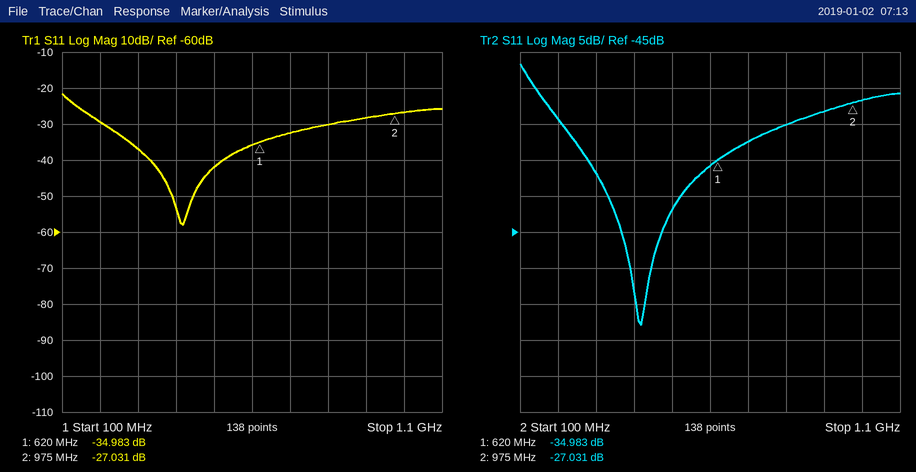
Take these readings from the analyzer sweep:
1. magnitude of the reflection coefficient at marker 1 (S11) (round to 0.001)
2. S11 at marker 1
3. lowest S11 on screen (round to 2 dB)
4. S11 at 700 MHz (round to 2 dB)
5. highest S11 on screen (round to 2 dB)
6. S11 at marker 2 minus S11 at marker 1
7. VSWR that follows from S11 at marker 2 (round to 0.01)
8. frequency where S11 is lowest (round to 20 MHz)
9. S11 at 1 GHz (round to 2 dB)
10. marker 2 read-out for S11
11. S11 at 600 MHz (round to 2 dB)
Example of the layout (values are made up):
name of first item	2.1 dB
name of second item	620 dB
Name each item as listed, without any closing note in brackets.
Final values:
magnitude of the reflection coefficient at marker 1 (S11)	0.018
S11 at marker 1	-34.983 dB
lowest S11 on screen	-58 dB
S11 at 700 MHz	-32 dB
highest S11 on screen	-22 dB
S11 at marker 2 minus S11 at marker 1	7.952 dB
VSWR that follows from S11 at marker 2	1.09
frequency where S11 is lowest	420 MHz
S11 at 1 GHz	-26 dB
marker 2 read-out for S11	-27.031 dB
S11 at 600 MHz	-36 dB
